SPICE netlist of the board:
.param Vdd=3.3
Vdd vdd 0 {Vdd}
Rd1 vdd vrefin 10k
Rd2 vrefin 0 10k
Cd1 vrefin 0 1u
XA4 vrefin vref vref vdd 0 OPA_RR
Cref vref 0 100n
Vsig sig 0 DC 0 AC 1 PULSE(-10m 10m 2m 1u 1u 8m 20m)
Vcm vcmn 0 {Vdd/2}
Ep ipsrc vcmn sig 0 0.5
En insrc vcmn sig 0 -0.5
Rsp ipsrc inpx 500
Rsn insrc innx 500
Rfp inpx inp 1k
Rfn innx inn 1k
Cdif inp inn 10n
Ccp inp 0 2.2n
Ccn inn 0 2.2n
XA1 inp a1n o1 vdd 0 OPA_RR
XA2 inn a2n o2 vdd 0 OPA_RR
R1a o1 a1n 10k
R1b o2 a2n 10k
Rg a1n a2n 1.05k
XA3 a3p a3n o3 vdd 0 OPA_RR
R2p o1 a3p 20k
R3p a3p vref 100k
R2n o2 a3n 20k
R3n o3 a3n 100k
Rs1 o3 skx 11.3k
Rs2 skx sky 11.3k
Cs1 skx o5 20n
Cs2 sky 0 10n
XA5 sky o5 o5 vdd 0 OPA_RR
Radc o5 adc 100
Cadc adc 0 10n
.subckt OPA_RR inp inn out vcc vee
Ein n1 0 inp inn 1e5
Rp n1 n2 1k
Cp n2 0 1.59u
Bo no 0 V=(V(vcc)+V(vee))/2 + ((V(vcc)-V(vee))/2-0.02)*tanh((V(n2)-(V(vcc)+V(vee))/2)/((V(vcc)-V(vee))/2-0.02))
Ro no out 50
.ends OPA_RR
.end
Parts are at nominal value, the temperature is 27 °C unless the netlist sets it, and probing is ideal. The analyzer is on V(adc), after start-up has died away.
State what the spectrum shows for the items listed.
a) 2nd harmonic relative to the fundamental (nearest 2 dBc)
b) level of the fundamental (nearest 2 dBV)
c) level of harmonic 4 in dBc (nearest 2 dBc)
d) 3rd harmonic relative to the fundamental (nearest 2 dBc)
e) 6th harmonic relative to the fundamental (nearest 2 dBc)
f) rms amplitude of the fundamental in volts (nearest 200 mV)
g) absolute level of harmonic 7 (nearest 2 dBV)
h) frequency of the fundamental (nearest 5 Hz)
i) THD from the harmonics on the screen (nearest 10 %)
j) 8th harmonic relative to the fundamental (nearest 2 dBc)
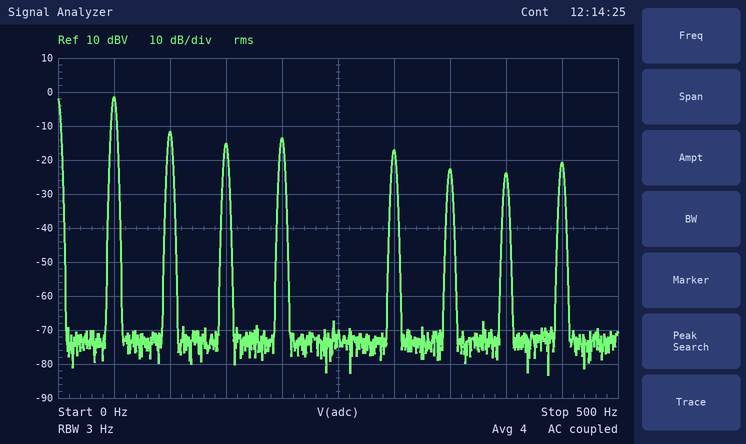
-10 dBc
-2 dBV
-12 dBc
-14 dBc
-16 dBc
800 mV
-22 dBV
50 Hz
50 %
-22 dBc
